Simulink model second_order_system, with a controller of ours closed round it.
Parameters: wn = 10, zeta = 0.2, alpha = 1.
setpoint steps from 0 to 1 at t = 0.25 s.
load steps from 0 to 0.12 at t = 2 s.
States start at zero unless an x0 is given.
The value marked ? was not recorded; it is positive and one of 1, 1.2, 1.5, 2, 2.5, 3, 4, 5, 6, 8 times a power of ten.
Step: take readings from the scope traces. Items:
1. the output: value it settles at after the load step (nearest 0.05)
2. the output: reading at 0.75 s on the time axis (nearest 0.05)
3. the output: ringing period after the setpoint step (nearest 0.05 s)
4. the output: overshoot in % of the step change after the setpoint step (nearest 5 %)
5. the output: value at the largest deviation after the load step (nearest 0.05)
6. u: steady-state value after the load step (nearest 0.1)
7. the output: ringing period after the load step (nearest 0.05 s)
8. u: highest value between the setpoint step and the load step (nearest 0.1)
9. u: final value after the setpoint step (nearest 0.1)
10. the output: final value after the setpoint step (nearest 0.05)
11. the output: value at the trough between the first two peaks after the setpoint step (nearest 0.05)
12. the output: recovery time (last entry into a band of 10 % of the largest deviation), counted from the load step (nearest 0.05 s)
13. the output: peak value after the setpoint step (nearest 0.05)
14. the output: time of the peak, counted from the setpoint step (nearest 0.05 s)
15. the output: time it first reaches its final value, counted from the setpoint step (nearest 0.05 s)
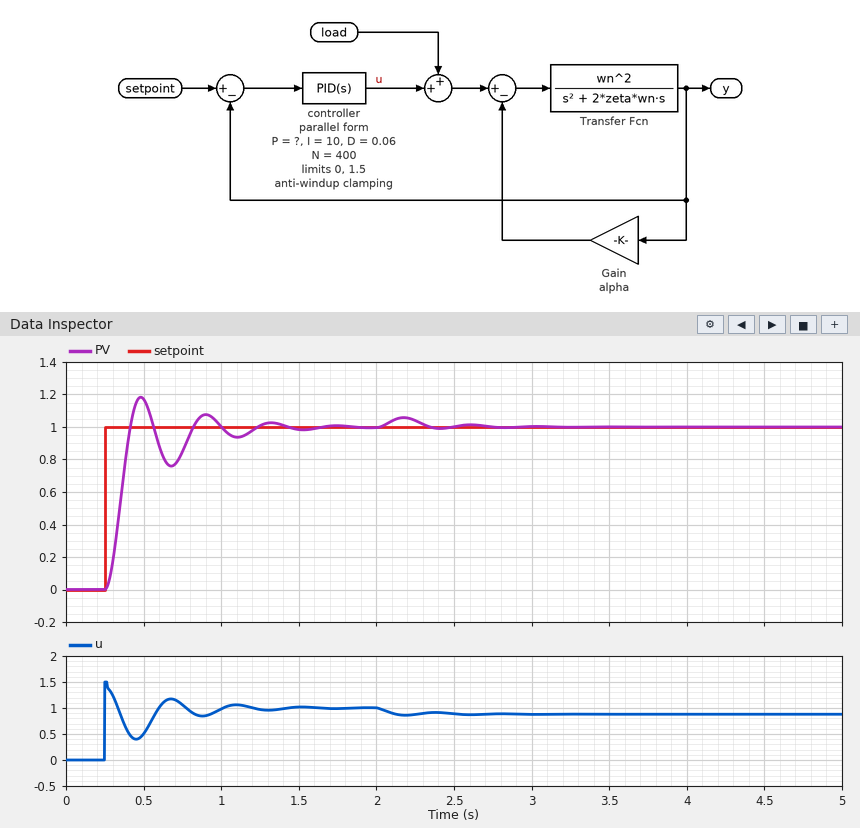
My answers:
1.00
0.85
0.40 s
20 %
1.05
0.9
0.45 s
1.5
1.0
1.00
0.75
0.70 s
1.20
0.25 s
0.15 s
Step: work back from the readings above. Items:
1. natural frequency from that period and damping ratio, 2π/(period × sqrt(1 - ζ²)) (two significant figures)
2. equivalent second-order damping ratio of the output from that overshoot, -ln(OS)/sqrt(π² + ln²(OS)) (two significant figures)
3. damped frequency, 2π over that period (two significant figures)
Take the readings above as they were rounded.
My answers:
18 rad/s
0.46
16 rad/s
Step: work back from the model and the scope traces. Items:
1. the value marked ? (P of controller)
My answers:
1.5
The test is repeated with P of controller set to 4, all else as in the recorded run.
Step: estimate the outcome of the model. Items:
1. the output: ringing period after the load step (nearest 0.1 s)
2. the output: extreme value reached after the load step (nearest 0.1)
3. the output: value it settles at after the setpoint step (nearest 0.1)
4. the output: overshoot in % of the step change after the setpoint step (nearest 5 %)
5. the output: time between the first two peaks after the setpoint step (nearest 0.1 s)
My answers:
0.3 s
1.0
1.0
15 %
0.3 s
